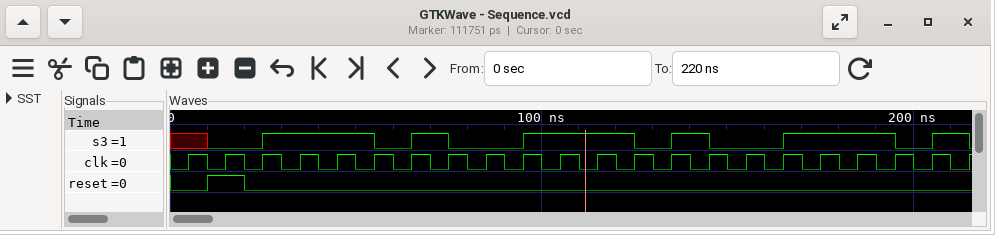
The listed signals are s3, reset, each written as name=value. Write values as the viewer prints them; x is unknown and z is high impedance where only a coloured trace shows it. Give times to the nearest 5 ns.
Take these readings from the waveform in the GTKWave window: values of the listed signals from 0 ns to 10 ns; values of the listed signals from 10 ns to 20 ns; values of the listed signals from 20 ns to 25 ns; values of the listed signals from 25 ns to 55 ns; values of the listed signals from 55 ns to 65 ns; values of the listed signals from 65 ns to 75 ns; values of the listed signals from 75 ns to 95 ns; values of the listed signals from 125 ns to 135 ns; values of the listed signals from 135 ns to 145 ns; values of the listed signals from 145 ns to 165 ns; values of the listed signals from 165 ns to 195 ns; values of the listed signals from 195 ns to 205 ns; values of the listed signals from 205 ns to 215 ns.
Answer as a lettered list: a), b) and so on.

a) s3=x, reset=0
b) s3=0, reset=1
c) s3=0, reset=0
d) s3=1, reset=0
e) s3=0, reset=0
f) s3=1, reset=0
g) s3=0, reset=0
h) s3=0, reset=0
i) s3=1, reset=0
j) s3=0, reset=0
k) s3=1, reset=0
l) s3=0, reset=0
m) s3=1, reset=0
